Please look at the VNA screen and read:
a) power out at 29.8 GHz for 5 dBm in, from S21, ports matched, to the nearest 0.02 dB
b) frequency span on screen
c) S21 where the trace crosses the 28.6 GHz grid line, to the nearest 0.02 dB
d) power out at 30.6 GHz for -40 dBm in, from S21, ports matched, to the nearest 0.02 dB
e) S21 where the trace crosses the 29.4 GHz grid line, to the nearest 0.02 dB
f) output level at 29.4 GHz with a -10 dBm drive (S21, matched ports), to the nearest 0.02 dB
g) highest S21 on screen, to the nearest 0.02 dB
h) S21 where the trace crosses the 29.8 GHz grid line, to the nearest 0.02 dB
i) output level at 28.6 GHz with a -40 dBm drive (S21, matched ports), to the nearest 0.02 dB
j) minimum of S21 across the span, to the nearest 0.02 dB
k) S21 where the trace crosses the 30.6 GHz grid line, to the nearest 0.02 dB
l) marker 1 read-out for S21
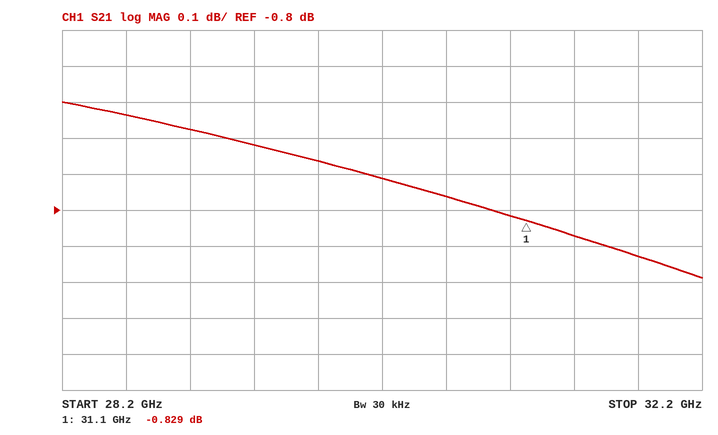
4.34 dBm
4 GHz
-0.54 dB
-40.76 dBm
-0.62 dB
-10.62 dBm
-0.50 dB
-0.66 dB
-40.54 dBm
-0.98 dB
-0.76 dB
-0.829 dB
